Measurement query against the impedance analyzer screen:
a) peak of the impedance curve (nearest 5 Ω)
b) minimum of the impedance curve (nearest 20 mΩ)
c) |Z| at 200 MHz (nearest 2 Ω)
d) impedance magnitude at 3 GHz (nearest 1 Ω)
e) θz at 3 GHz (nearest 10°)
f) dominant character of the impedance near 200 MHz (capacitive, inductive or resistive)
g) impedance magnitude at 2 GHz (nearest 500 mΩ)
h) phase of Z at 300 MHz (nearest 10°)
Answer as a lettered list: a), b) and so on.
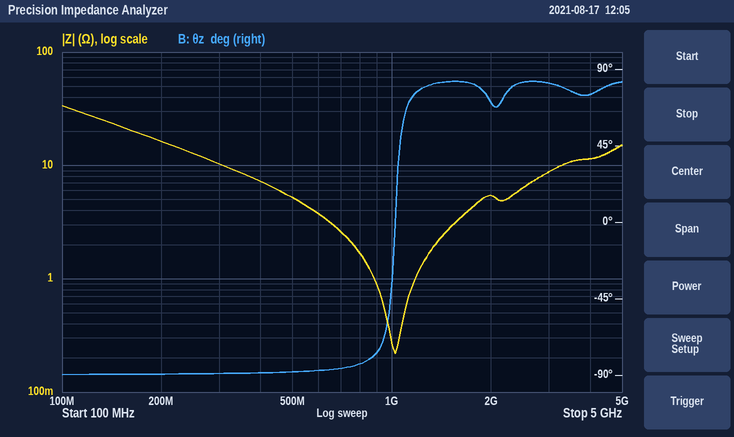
a) 35 Ω
b) 220 mΩ
c) 16 Ω
d) 9 Ω
e) 80°
f) capacitive
g) 5.5 Ω
h) -90°
